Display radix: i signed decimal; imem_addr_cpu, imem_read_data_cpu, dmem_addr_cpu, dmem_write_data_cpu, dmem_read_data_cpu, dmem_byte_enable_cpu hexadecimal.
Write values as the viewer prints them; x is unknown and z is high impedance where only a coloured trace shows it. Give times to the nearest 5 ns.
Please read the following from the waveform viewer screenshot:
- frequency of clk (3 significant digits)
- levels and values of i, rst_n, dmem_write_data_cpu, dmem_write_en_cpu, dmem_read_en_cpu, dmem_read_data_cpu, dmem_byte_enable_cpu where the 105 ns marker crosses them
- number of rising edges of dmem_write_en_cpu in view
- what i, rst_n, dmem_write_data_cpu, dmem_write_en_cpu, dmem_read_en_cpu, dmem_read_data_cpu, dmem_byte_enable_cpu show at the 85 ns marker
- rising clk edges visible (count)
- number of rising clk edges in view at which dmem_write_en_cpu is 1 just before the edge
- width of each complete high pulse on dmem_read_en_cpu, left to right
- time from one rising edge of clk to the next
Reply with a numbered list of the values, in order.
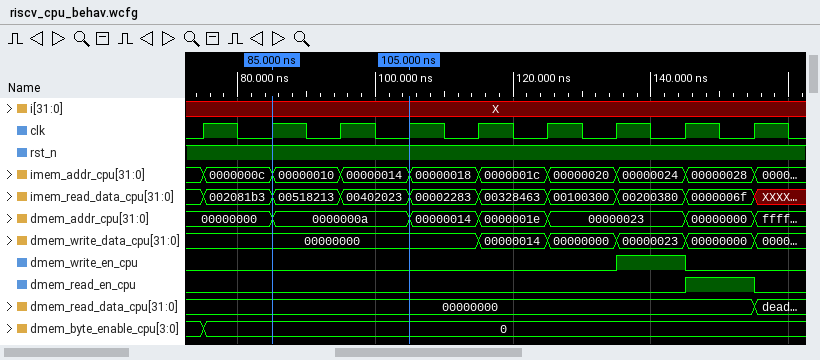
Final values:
1. 100 MHz
2. i=X, rst_n=1, dmem_write_data_cpu=00000000, dmem_write_en_cpu=0, dmem_read_en_cpu=0, dmem_read_data_cpu=00000000, dmem_byte_enable_cpu=0
3. 1
4. i=X, rst_n=1, dmem_write_data_cpu=00000000, dmem_write_en_cpu=0, dmem_read_en_cpu=0, dmem_read_data_cpu=00000000, dmem_byte_enable_cpu=0
5. 9
6. 1
7. 10 ns
8. 10 ns
